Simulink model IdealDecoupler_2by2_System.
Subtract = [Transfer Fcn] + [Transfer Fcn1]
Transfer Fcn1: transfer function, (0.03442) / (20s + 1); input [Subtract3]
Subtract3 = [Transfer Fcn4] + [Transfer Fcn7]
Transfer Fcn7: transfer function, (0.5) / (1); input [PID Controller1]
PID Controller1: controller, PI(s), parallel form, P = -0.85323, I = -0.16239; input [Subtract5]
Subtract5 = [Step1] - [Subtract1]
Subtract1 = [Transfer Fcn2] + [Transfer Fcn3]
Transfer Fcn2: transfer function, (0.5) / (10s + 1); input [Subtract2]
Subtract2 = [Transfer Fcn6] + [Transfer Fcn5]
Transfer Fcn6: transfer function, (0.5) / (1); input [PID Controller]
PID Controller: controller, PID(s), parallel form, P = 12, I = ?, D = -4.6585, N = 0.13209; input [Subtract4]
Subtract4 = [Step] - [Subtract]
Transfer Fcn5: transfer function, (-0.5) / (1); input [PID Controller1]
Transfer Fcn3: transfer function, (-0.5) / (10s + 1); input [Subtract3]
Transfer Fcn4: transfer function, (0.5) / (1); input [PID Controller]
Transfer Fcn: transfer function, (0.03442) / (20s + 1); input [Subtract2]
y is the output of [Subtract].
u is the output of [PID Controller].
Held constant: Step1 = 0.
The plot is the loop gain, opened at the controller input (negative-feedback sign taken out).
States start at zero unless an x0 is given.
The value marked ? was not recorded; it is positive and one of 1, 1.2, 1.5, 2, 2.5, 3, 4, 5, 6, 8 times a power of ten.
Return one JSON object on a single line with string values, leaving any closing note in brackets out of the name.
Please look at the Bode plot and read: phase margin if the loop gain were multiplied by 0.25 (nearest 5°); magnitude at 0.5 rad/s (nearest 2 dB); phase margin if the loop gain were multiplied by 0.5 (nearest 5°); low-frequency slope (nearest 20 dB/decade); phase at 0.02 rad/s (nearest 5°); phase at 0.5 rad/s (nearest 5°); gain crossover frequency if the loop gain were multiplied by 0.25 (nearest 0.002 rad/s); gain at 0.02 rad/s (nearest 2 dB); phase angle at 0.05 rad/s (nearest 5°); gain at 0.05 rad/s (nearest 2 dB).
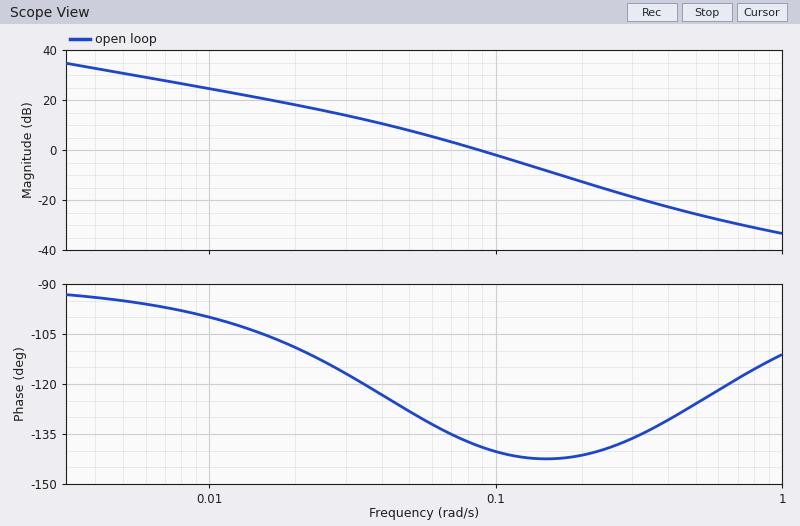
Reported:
{"phase margin if the loop gain were multiplied by 0.25": "60°", "magnitude at 0.5 rad/s": "-26 dB", "phase margin if the loop gain were multiplied by 0.5": "50°", "low-frequency slope": "-20 dB/decade", "phase at 0.02 rad/s": "-110°", "phase at 0.5 rad/s": "-125°", "gain crossover frequency if the loop gain were multiplied by 0.25": "0.036 rad/s", "gain at 0.02 rad/s": "18 dB", "phase angle at 0.05 rad/s": "-130°", "gain at 0.05 rad/s": "8 dB"}
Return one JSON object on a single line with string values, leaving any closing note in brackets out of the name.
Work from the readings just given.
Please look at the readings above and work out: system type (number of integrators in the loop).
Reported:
{"system type": "1"}
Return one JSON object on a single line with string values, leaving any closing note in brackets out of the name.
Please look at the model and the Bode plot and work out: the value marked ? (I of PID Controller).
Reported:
{"the value marked ?": "5"}
